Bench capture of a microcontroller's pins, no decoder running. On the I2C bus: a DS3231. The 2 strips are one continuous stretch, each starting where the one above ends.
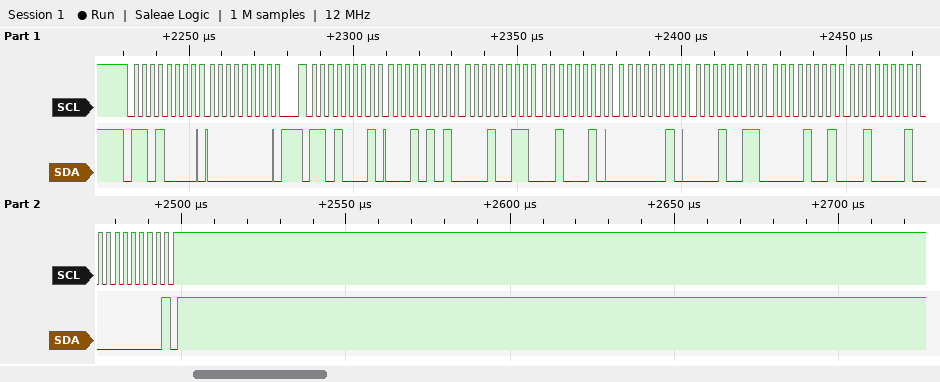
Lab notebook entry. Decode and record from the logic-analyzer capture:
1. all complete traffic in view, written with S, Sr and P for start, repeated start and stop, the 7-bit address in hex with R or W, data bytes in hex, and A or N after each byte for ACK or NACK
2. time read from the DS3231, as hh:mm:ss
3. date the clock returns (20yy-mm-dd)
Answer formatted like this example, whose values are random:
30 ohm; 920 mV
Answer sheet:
S 68W A 00 A Sr 68R A 15 A 13 A 22 A 02 A 13 A 09 A 21 A 00 N P; 22:13:15; 2021-09-13
